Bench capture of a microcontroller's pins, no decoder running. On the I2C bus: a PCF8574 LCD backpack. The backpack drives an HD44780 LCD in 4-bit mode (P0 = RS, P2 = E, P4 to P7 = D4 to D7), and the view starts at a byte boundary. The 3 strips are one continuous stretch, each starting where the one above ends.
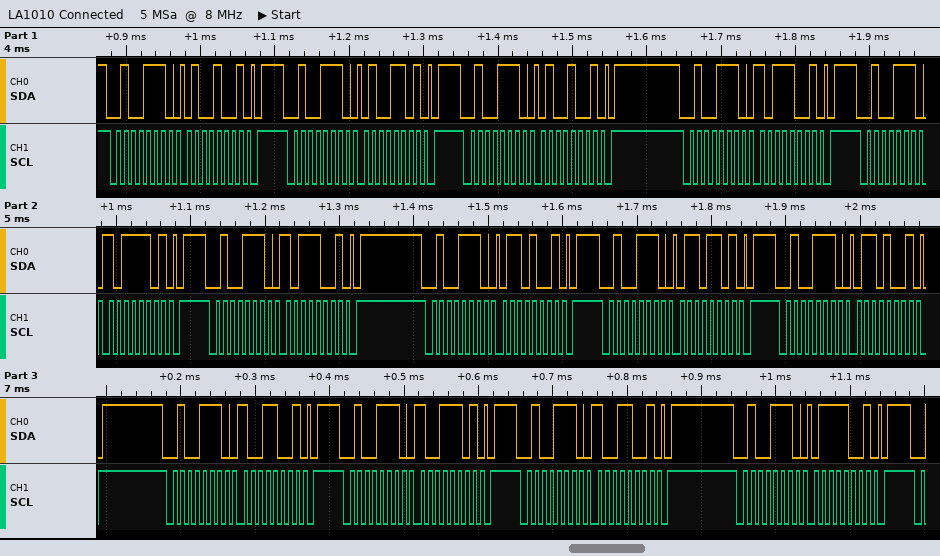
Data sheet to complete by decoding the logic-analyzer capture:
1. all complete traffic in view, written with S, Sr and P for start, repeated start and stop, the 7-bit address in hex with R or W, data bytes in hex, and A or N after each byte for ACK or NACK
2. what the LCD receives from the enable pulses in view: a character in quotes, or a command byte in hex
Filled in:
S 27W A 49 A P S 27W A 4D A P S 27W A 49 A P S 27W A B9 A P S 27W A BD A P S 27W A B9 A P S 27W A 69 A P S 27W A 6D A P S 27W A 69 A P S 27W A 99 A P S 27W A 9D A P S 27W A 99 A P S 27W A 79 A P
'K' 'i'
